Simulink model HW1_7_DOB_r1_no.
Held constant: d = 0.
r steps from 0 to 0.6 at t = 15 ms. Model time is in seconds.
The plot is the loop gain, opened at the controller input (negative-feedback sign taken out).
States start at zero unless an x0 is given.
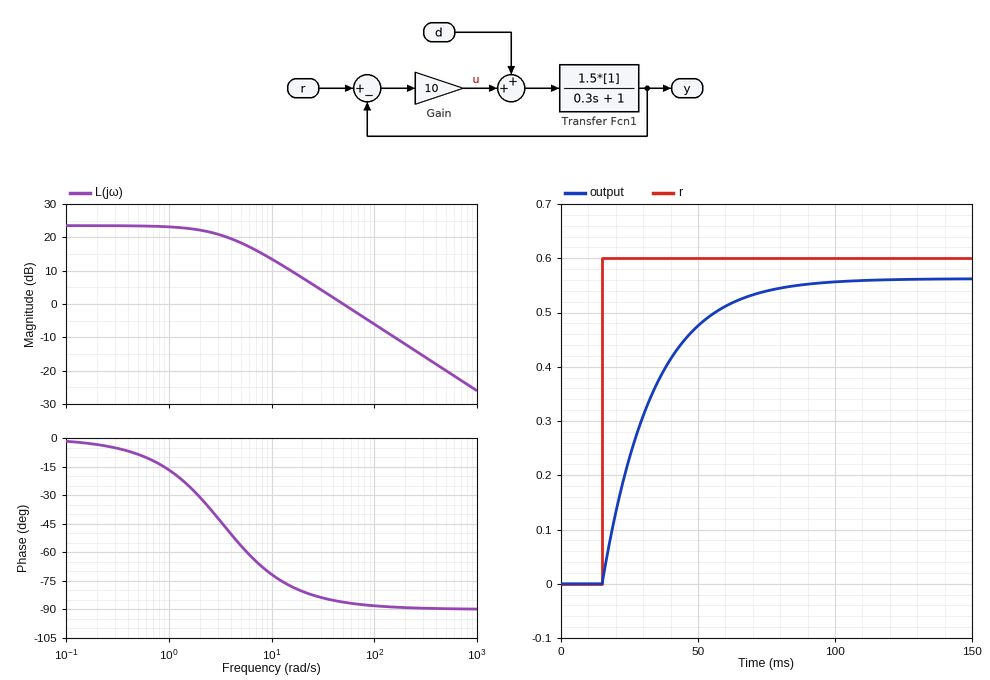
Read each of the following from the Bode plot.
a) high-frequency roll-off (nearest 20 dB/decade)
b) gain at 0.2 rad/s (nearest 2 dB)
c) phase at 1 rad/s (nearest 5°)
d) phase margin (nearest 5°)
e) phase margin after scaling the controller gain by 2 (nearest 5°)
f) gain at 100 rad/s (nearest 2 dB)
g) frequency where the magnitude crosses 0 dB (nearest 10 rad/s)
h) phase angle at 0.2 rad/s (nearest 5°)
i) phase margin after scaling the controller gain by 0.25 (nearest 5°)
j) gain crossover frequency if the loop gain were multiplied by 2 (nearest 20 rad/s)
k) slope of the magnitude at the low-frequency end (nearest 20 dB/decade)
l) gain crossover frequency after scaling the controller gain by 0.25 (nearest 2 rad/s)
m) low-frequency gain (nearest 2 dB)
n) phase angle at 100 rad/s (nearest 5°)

-20 dB/decade
24 dB
-15°
95°
90°
-6 dB
50 rad/s
-5°
105°
100 rad/s
0 dB/decade
12 rad/s
24 dB
-90°
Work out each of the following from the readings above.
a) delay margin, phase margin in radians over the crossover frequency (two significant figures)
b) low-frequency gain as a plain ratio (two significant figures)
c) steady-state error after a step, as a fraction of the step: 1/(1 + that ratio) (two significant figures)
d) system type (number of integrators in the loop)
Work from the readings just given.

0.033 s
16
0.059
0
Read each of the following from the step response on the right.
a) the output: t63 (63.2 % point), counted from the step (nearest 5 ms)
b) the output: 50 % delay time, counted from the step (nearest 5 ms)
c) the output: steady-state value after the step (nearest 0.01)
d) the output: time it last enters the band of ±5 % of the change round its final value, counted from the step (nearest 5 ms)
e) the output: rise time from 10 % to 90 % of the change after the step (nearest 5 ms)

20 ms
15 ms
0.56
55 ms
40 ms
